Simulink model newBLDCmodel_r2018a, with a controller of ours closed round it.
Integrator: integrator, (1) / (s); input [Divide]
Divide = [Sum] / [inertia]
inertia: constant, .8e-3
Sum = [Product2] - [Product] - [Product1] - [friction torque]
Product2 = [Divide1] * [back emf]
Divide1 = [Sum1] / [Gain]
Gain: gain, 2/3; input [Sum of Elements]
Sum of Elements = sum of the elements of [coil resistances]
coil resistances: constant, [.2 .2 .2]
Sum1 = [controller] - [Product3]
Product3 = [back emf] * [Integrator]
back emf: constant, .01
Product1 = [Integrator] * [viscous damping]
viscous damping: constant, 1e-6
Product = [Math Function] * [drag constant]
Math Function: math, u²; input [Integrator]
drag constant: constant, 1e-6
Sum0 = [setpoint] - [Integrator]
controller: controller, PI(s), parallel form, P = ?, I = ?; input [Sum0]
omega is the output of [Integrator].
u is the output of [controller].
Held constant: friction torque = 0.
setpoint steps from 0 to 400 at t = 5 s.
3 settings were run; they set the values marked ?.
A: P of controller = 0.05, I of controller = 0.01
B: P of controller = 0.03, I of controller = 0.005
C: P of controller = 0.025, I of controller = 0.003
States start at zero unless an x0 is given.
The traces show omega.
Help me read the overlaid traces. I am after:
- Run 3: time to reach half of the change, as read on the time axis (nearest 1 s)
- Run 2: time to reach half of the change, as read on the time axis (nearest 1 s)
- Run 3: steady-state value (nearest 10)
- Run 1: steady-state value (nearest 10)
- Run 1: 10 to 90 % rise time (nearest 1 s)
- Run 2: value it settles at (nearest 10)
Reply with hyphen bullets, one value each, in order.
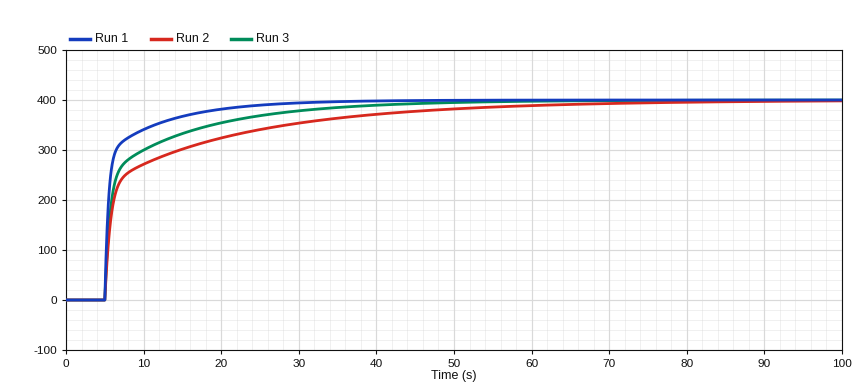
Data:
- 6 s
- 6 s
- 400
- 400
- 8 s
- 400
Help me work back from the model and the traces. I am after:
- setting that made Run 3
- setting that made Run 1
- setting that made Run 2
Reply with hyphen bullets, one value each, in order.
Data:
- B
- A
- C
